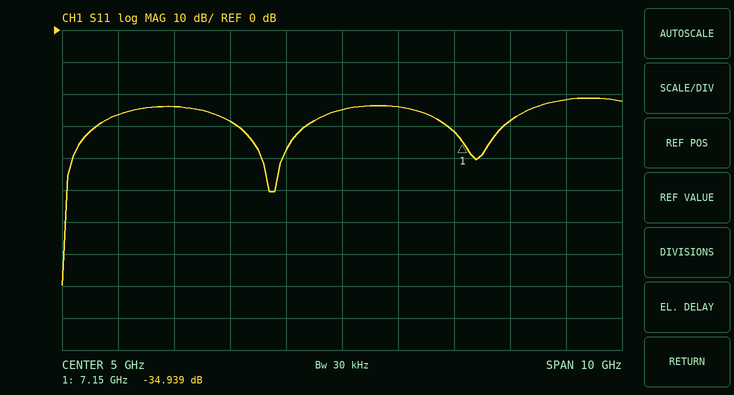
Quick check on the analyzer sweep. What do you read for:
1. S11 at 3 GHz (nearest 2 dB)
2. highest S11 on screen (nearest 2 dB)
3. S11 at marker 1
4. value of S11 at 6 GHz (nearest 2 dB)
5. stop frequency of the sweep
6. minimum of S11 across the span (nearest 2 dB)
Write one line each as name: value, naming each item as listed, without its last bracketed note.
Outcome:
S11 at 3 GHz: -28 dB
highest S11 on screen: -22 dB
S11 at marker 1: -34.939 dB
value of S11 at 6 GHz: -24 dB
stop frequency of the sweep: 10 GHz
minimum of S11 across the span: -80 dB
